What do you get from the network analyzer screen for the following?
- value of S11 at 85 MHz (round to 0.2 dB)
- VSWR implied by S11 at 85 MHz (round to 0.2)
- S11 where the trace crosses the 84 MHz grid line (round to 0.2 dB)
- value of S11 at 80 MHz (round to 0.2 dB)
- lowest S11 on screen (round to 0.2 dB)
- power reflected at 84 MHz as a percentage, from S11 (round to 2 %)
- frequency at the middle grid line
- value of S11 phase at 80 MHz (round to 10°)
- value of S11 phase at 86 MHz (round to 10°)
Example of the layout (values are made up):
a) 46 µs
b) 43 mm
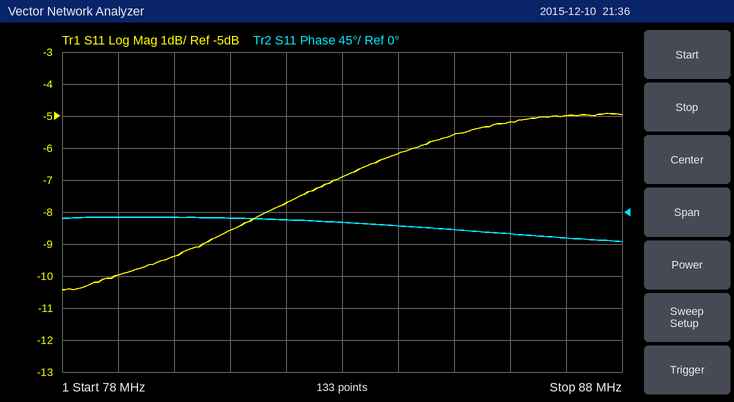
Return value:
a) -5.6 dB
b) 3.2
c) -6.2 dB
d) -9.4 dB
e) -10.4 dB
f) 24 %
g) 83 MHz
h) -10°
i) -30°
